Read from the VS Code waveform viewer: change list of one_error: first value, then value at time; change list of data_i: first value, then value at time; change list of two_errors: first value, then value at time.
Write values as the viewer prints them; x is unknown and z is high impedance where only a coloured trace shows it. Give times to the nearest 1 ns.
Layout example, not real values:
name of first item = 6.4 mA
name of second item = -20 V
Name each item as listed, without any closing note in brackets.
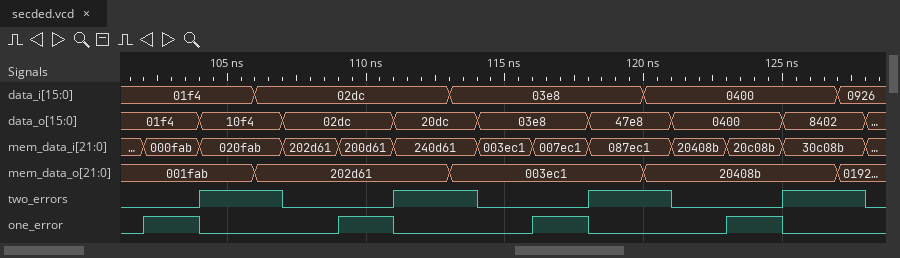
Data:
change list of one_error: first value, then value at time = 0, 1 at 102 ns, 0 at 104 ns, 1 at 109 ns, 0 at 111 ns, 1 at 116 ns, 0 at 118 ns, 1 at 123 ns, 0 at 125 ns
change list of data_i: first value, then value at time = 01f4, 02dc at 106 ns, 03e8 at 113 ns, 0400 at 120 ns, 0926 at 127 ns
change list of two_errors: first value, then value at time = 0, 1 at 104 ns, 0 at 107 ns, 1 at 111 ns, 0 at 114 ns, 1 at 118 ns, 0 at 121 ns, 1 at 125 ns, 0 at 128 ns
